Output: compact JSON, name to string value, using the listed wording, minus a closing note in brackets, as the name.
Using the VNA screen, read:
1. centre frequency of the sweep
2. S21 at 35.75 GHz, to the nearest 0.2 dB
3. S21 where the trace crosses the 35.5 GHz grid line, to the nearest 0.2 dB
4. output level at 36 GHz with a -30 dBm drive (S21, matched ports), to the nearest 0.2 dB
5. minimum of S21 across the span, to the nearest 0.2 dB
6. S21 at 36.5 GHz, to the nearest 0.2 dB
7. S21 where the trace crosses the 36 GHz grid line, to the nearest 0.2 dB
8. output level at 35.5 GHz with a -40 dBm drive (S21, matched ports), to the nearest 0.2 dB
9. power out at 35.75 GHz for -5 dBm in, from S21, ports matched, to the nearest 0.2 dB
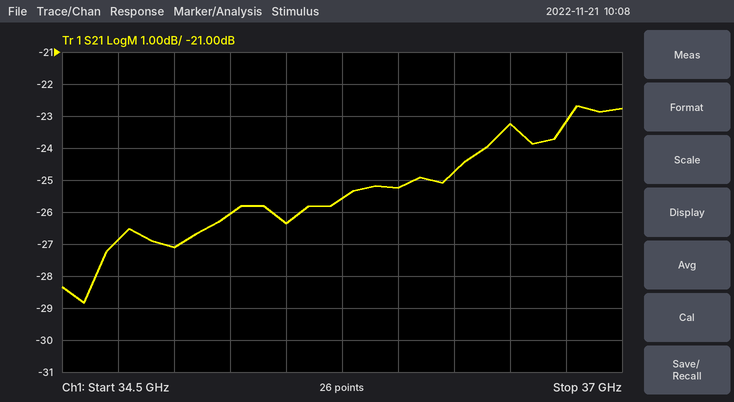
{"centre frequency of the sweep": "35.75 GHz", "S21 at 35.75 GHz, to the nearest 0.2 dB": "-25.6 dB", "S21 where the trace crosses the 35.5 GHz grid line, to the nearest 0.2 dB": "-26.4 dB", "output level at 36 GHz with a -30 dBm drive (S21, matched ports), to the nearest 0.2 dB": "-55.2 dBm", "minimum of S21 across the span, to the nearest 0.2 dB": "-28.8 dB", "S21 at 36.5 GHz, to the nearest 0.2 dB": "-23.2 dB", "S21 where the trace crosses the 36 GHz grid line, to the nearest 0.2 dB": "-25.2 dB", "output level at 35.5 GHz with a -40 dBm drive (S21, matched ports), to the nearest 0.2 dB": "-66.4 dBm", "power out at 35.75 GHz for -5 dBm in, from S21, ports matched, to the nearest 0.2 dB": "-30.6 dBm"}
